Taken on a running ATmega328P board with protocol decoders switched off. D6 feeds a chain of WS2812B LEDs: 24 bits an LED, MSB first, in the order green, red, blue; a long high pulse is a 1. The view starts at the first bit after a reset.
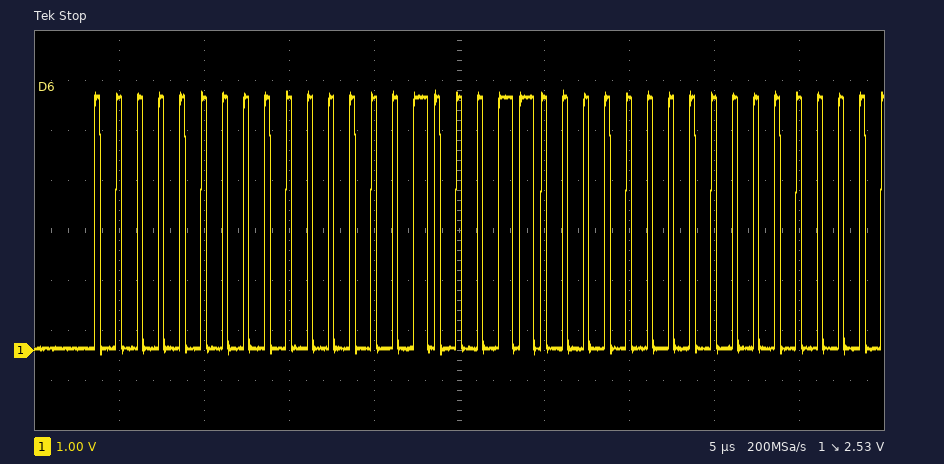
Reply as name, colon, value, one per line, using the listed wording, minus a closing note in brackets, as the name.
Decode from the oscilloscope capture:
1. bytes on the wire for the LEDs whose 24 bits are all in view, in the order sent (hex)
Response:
bytes on the wire for the LEDs whose 24 bits are all in view, in the order sent: 00 01 18
